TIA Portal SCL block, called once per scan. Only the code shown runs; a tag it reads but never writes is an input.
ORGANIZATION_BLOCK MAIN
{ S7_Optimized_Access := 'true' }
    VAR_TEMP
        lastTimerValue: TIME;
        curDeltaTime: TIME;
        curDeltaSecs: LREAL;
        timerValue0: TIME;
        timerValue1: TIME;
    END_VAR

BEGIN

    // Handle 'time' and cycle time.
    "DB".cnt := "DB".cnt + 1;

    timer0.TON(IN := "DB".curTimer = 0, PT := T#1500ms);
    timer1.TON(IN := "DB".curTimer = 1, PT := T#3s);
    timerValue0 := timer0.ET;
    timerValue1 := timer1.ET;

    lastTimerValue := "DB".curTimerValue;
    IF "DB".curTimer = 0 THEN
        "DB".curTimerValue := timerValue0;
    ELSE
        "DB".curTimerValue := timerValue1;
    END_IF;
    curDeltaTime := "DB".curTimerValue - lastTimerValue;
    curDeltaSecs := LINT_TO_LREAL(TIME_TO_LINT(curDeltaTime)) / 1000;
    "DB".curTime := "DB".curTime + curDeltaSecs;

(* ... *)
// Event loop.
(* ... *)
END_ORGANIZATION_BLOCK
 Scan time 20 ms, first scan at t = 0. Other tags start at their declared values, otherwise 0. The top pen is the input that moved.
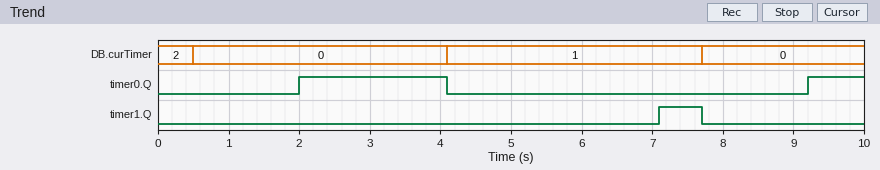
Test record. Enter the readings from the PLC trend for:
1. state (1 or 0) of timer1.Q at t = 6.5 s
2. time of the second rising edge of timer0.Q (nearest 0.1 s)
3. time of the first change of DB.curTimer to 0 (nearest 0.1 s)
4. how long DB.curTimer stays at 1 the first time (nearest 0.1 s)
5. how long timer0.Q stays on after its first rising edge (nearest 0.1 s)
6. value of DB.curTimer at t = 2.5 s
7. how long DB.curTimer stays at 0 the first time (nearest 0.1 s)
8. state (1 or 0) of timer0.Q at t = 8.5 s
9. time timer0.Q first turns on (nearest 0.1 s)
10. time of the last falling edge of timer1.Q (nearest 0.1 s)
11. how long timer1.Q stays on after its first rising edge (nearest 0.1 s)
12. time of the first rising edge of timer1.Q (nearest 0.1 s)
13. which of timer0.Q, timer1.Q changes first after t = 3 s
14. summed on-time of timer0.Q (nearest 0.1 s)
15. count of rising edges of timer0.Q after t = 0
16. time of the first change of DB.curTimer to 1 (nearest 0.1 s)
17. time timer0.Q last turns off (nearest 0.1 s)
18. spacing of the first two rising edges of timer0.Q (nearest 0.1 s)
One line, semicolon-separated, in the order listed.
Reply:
0; 9.2 s; 0.5 s; 3.6 s; 2.1 s; 0; 3.6 s; 0; 2.0 s; 7.7 s; 0.6 s; 7.1 s; timer0.Q; 2.9 s; 2; 4.1 s; 4.1 s; 7.2 s
